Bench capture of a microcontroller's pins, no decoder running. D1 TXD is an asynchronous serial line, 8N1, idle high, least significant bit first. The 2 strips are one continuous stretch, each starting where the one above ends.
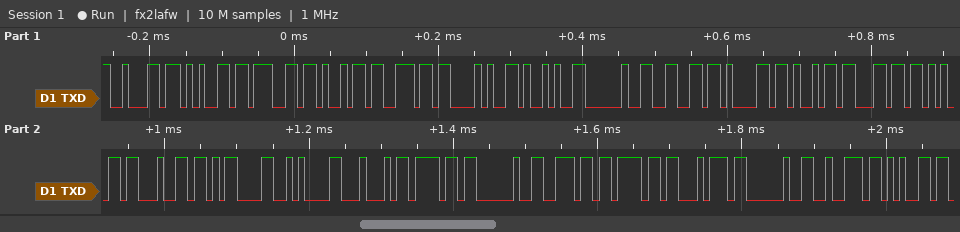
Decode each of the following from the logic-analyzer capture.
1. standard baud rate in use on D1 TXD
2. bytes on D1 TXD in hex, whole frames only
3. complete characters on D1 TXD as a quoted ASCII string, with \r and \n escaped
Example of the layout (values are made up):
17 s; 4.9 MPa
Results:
115200 baud; 62 65 67 69 6E 28 29 20 66 61 69 6C 65 64 0D 0A 44 6F 20 6E 6F 74 20 72 65; "begin() failed\r\nDo not re"
